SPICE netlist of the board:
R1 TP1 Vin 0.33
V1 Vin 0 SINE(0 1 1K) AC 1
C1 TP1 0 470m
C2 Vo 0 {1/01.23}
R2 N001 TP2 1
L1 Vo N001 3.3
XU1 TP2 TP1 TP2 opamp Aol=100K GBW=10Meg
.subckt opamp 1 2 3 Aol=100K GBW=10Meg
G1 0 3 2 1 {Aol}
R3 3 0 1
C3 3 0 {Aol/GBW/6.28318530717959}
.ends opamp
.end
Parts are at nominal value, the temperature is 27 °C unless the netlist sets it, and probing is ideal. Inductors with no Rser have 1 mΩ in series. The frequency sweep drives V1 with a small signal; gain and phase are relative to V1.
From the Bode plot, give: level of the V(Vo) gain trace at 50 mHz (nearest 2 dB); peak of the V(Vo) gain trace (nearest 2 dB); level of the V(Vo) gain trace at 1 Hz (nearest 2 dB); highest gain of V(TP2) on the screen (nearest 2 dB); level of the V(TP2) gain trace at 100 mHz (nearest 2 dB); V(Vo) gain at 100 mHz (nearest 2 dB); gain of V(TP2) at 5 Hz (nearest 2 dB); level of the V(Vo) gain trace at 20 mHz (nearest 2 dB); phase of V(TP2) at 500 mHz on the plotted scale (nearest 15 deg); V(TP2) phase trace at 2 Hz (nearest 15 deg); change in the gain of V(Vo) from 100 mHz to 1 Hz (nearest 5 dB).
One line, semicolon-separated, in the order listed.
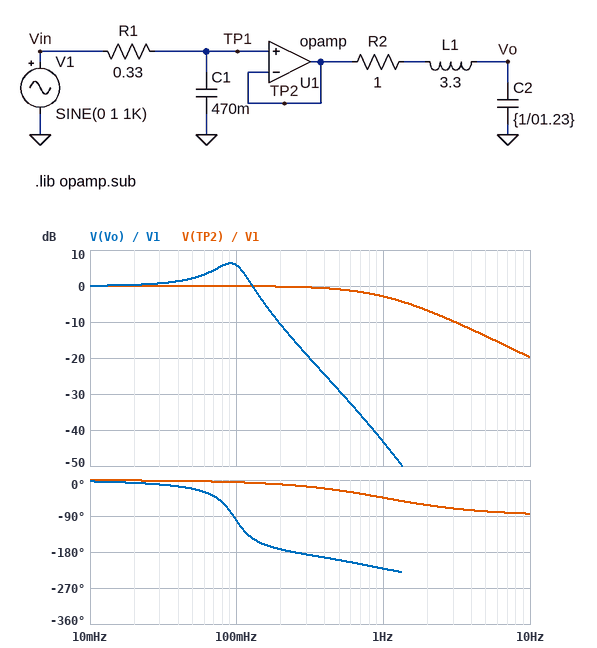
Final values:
2 dB; 6 dB; -44 dB; 0 dB; 0 dB; 6 dB; -14 dB; 0 dB; -30 deg; -60 deg; -50 dB
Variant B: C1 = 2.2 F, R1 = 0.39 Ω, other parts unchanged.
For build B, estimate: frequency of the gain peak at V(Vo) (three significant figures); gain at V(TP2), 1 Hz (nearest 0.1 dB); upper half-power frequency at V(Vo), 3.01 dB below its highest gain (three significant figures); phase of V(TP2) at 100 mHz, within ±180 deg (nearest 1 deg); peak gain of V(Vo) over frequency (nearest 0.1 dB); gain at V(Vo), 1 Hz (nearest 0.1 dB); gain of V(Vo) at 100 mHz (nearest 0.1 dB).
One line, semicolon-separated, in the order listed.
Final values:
89.6 mHz; -14.8 dB; 111 mHz; -28 deg; 5.4 dB; -55.2 dB; 4.7 dB
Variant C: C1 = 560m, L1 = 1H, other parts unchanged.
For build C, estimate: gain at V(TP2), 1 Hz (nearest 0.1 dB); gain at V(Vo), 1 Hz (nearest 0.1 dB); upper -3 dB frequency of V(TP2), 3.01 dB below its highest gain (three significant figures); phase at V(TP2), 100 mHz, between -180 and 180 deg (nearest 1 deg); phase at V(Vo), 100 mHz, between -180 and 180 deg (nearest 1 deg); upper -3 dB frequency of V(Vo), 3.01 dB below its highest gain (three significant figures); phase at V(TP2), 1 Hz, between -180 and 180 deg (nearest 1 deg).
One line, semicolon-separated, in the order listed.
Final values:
-3.7 dB; -33.7 dB; 861 mHz; -7 deg; -44 deg; 207 mHz; -49 deg
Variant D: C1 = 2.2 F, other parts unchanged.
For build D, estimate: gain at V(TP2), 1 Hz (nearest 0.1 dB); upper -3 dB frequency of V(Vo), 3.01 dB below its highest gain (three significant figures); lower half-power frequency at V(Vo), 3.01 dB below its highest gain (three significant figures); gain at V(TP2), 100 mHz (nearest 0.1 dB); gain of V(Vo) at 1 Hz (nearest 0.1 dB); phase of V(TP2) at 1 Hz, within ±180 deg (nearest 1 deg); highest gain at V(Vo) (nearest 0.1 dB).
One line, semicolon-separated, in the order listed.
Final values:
-13.4 dB; 112 mHz; 57.6 mHz; -0.8 dB; -53.8 dB; -78 deg; 5.7 dB
